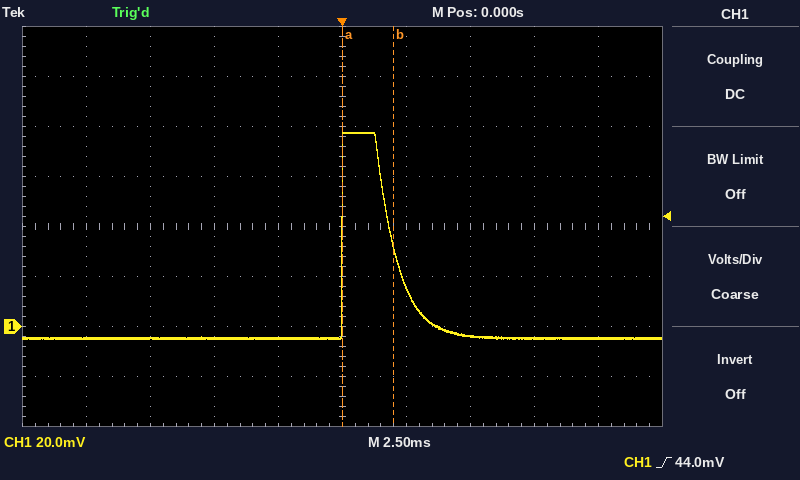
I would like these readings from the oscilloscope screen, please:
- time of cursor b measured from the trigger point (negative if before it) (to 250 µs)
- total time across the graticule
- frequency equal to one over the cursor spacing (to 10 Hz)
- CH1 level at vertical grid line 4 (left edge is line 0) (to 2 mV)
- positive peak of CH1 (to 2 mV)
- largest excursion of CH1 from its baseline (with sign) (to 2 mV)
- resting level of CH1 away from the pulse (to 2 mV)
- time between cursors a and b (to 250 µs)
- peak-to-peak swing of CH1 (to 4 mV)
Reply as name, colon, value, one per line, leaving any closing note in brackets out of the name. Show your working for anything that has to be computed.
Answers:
time of cursor b measured from the trigger point (negative if before it): +2.00 ms
total time across the graticule: 25 ms
frequency equal to one over the cursor spacing: 1 / 2.00 ms ≈ 500 Hz
CH1 level at vertical grid line 4 (left edge is line 0): -4 mV
positive peak of CH1: 78 mV
largest excursion of CH1 from its baseline (with sign): 78 mV − (-4 mV) = +82 mV
resting level of CH1 away from the pulse: -4 mV
time between cursors a and b: 2.00 ms
peak-to-peak swing of CH1: 84 mV
